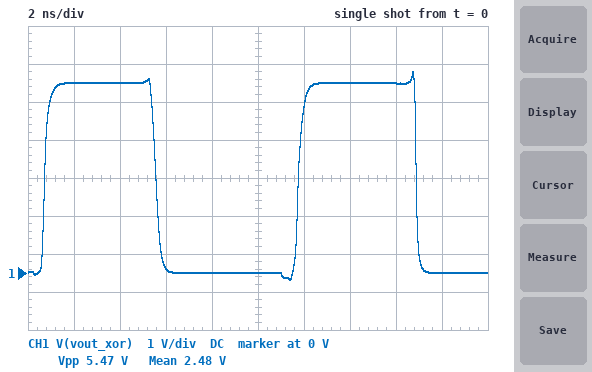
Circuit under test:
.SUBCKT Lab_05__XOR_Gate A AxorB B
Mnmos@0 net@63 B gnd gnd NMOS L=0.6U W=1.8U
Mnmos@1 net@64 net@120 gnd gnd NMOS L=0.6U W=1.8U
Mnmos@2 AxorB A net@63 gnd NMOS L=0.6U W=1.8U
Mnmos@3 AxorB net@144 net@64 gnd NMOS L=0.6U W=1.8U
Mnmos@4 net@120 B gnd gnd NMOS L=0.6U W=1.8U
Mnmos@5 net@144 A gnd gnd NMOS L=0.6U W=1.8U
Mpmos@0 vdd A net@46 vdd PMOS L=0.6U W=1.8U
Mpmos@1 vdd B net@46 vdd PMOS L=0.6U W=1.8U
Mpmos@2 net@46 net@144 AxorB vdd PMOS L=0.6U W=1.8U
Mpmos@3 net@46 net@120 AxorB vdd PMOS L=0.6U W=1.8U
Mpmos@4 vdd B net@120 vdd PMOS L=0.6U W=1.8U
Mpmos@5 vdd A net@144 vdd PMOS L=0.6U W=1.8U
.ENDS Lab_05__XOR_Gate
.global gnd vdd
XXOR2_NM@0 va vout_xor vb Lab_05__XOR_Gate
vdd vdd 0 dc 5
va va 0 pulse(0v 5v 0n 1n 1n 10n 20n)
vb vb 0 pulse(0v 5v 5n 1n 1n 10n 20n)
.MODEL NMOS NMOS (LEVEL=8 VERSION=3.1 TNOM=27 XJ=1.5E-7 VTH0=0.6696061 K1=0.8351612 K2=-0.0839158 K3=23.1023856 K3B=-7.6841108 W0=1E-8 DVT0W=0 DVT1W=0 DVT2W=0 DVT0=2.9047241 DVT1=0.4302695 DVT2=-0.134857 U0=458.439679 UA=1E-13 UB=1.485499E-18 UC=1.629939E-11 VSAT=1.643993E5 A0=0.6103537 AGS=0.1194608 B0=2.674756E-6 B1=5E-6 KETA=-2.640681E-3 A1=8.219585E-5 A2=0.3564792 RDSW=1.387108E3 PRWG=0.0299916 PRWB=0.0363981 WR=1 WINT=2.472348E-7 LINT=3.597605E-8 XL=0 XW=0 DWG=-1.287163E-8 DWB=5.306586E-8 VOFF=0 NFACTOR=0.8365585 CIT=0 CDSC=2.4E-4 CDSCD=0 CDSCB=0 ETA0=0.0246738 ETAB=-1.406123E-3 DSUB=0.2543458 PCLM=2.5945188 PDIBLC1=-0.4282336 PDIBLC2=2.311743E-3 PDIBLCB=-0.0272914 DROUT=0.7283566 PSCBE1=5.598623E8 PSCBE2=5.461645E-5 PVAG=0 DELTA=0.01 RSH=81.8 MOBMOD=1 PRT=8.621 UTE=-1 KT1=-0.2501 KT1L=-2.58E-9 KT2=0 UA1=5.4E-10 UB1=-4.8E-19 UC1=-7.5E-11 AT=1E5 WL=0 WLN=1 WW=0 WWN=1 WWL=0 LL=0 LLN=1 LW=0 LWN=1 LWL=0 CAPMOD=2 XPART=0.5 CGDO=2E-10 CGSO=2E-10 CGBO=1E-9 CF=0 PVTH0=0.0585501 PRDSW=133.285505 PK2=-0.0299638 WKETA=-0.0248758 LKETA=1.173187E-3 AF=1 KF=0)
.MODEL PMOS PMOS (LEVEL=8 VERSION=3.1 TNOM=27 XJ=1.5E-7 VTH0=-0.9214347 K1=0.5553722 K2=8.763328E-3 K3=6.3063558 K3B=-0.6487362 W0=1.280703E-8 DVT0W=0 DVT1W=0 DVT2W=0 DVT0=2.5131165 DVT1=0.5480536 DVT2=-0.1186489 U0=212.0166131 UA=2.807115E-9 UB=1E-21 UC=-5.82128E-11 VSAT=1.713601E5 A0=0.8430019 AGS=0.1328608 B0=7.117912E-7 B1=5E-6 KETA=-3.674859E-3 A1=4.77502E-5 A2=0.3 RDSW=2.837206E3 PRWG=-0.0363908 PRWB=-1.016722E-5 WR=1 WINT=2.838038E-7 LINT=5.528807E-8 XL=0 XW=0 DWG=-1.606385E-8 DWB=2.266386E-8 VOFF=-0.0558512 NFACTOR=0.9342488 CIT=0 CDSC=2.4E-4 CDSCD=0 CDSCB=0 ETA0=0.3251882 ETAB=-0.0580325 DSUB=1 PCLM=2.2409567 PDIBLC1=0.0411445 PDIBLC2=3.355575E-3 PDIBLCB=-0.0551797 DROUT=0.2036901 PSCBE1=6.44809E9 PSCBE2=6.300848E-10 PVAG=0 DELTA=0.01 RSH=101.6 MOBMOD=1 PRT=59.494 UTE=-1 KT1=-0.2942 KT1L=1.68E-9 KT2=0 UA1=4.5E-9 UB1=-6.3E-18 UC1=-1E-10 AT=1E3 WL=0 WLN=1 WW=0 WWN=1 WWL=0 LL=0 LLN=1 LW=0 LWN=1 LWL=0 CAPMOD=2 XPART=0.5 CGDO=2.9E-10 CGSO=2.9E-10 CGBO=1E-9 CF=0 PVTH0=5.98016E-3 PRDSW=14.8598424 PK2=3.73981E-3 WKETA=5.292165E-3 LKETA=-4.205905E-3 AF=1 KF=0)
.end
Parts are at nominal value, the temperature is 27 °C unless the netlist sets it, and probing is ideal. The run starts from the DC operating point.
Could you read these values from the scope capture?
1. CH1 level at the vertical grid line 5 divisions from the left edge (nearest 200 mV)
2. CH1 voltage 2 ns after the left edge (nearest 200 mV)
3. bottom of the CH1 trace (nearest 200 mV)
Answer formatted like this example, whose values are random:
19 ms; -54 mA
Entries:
0 V; 5.0 V; -200 mV
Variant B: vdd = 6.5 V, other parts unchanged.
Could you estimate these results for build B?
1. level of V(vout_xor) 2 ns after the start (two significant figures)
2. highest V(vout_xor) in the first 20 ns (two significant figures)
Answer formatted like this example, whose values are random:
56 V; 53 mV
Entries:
6.5 V; 6.7 V
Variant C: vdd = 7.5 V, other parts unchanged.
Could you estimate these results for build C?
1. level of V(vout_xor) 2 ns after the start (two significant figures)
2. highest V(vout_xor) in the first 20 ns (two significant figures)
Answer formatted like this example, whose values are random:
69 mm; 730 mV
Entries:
7.5 V; 7.6 V
